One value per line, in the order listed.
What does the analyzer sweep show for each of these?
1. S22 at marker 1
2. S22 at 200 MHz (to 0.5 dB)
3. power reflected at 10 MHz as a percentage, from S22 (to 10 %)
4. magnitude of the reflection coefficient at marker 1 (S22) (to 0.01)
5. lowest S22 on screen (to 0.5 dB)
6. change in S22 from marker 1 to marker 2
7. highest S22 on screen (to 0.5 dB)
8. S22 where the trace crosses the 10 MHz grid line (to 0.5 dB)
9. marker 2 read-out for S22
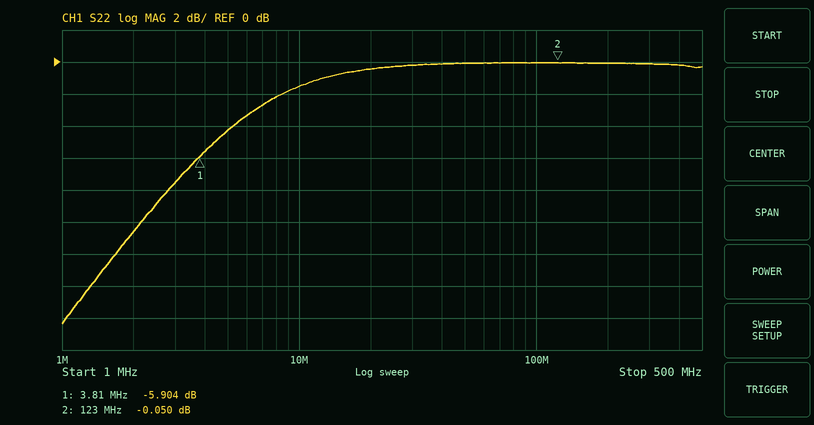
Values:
-5.904 dB
0.0 dB
70 %
0.51
-16.5 dB
5.854 dB
0.0 dB
-1.5 dB
-0.050 dB
